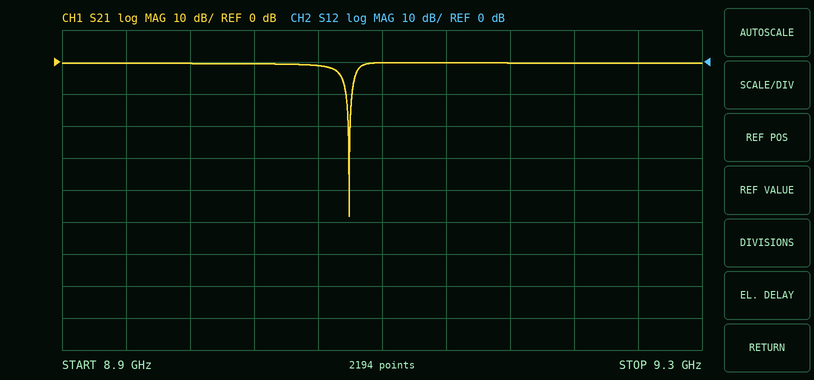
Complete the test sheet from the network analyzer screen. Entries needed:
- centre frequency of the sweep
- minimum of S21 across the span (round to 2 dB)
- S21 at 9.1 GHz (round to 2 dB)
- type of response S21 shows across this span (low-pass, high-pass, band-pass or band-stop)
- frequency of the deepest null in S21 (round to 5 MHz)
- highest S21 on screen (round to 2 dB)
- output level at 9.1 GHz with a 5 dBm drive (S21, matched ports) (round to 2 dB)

9.1 GHz
-48 dB
0 dB
band-stop
9.080 GHz
0 dB
4 dBm
